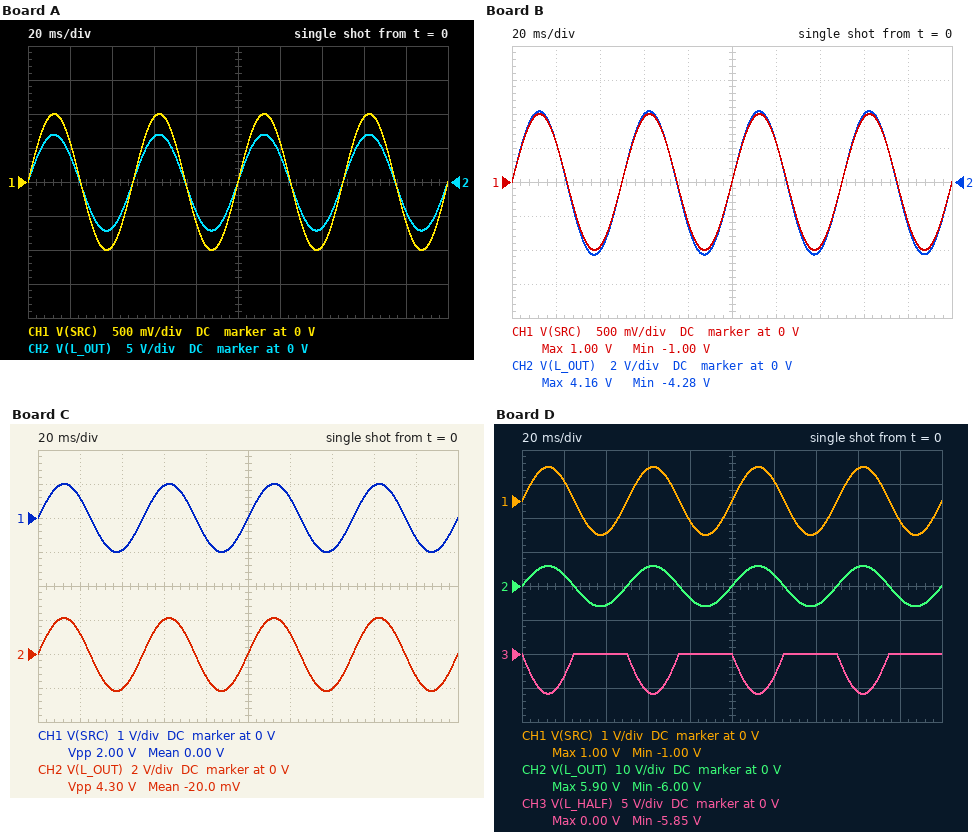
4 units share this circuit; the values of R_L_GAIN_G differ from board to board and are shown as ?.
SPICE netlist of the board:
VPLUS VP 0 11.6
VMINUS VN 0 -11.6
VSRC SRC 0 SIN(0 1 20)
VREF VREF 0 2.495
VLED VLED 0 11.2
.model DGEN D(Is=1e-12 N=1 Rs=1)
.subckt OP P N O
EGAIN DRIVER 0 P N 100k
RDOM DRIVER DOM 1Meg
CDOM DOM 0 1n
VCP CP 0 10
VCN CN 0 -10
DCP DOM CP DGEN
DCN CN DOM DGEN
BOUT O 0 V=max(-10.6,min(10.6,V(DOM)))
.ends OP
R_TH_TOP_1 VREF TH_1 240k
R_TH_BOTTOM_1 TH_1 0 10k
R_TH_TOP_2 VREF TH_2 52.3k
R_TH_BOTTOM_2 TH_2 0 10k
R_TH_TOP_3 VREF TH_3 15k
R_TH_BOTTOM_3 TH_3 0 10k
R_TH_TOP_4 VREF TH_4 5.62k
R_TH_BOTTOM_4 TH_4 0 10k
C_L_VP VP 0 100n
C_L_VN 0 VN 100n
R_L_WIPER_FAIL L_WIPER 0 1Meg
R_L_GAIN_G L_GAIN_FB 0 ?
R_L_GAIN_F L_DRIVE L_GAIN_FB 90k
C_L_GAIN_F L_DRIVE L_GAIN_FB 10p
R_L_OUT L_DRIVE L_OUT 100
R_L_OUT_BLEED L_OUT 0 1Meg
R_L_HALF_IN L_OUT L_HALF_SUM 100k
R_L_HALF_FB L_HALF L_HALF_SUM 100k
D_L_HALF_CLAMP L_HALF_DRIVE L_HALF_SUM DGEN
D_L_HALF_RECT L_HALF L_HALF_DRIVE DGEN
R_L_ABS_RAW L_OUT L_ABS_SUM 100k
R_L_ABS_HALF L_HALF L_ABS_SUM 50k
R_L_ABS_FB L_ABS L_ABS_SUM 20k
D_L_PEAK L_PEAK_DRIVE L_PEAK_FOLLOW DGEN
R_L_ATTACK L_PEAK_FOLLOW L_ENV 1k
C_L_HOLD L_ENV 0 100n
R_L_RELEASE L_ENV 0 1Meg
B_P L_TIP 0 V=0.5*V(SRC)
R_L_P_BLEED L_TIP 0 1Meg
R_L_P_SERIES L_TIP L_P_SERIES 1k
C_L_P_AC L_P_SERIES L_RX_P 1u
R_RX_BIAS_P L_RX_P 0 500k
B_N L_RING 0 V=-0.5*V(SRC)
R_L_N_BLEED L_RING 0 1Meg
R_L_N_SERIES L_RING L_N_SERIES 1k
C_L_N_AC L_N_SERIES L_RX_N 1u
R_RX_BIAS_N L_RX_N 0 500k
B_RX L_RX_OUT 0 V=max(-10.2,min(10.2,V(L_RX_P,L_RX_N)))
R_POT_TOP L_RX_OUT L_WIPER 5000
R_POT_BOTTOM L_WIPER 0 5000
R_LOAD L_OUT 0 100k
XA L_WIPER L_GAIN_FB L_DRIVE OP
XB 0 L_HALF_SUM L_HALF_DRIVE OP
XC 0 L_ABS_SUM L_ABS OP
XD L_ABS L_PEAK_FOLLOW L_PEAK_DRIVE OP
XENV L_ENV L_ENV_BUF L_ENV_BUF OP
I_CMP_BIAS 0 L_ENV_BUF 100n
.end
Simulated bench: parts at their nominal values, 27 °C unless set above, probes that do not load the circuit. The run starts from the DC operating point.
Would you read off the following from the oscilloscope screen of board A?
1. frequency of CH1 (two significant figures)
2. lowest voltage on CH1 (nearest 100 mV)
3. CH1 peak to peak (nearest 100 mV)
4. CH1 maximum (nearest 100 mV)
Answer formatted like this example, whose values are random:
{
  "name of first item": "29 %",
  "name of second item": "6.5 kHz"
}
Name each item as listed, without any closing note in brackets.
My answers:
{
  "frequency of CH1": "20 Hz",
  "lowest voltage on CH1": "-1.0 V",
  "CH1 peak to peak": "2.0 V",
  "CH1 maximum": "1.0 V"
}
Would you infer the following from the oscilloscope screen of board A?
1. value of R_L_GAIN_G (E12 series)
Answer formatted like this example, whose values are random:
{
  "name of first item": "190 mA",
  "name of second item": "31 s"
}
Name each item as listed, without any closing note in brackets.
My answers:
{
  "value of R_L_GAIN_G": "6.8 kΩ"
}
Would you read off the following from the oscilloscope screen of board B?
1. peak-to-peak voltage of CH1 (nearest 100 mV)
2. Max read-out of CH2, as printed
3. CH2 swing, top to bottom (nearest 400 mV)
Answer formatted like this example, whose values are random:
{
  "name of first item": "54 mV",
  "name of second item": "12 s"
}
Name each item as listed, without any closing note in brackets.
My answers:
{
  "peak-to-peak voltage of CH1": "2.0 V",
  "Max read-out of CH2, as printed": "4.16 V",
  "CH2 swing, top to bottom": "8.4 V"
}
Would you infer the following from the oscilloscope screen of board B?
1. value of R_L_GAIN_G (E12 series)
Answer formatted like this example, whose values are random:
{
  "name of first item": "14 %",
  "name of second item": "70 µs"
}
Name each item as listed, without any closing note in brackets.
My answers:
{
  "value of R_L_GAIN_G": "12 kΩ"
}
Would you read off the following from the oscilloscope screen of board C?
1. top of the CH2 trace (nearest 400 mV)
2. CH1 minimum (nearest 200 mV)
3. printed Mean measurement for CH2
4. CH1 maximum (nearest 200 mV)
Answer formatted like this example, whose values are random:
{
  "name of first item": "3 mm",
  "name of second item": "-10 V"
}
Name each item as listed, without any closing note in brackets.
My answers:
{
  "top of the CH2 trace": "2.0 V",
  "CH1 minimum": "-1.0 V",
  "printed Mean measurement for CH2": "-20.0 mV",
  "CH1 maximum": "1.0 V"
}
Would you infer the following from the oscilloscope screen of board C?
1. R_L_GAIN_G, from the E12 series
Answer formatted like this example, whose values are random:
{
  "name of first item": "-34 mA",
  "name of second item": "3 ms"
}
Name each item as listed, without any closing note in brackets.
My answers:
{
  "R_L_GAIN_G, from the E12 series": "27 kΩ"
}
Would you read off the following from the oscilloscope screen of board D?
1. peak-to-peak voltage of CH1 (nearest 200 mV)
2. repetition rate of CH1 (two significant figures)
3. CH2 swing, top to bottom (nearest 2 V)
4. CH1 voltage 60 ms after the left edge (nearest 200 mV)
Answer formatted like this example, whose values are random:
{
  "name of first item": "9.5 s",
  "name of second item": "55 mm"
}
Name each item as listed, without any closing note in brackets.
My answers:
{
  "peak-to-peak voltage of CH1": "2.0 V",
  "repetition rate of CH1": "20 Hz",
  "CH2 swing, top to bottom": "12 V",
  "CH1 voltage 60 ms after the left edge": "1.0 V"
}
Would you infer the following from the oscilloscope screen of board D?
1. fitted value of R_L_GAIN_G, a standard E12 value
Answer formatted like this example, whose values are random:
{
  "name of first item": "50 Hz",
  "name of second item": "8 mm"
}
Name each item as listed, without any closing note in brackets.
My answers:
{
  "fitted value of R_L_GAIN_G, a standard E12 value": "8.2 kΩ"
}
